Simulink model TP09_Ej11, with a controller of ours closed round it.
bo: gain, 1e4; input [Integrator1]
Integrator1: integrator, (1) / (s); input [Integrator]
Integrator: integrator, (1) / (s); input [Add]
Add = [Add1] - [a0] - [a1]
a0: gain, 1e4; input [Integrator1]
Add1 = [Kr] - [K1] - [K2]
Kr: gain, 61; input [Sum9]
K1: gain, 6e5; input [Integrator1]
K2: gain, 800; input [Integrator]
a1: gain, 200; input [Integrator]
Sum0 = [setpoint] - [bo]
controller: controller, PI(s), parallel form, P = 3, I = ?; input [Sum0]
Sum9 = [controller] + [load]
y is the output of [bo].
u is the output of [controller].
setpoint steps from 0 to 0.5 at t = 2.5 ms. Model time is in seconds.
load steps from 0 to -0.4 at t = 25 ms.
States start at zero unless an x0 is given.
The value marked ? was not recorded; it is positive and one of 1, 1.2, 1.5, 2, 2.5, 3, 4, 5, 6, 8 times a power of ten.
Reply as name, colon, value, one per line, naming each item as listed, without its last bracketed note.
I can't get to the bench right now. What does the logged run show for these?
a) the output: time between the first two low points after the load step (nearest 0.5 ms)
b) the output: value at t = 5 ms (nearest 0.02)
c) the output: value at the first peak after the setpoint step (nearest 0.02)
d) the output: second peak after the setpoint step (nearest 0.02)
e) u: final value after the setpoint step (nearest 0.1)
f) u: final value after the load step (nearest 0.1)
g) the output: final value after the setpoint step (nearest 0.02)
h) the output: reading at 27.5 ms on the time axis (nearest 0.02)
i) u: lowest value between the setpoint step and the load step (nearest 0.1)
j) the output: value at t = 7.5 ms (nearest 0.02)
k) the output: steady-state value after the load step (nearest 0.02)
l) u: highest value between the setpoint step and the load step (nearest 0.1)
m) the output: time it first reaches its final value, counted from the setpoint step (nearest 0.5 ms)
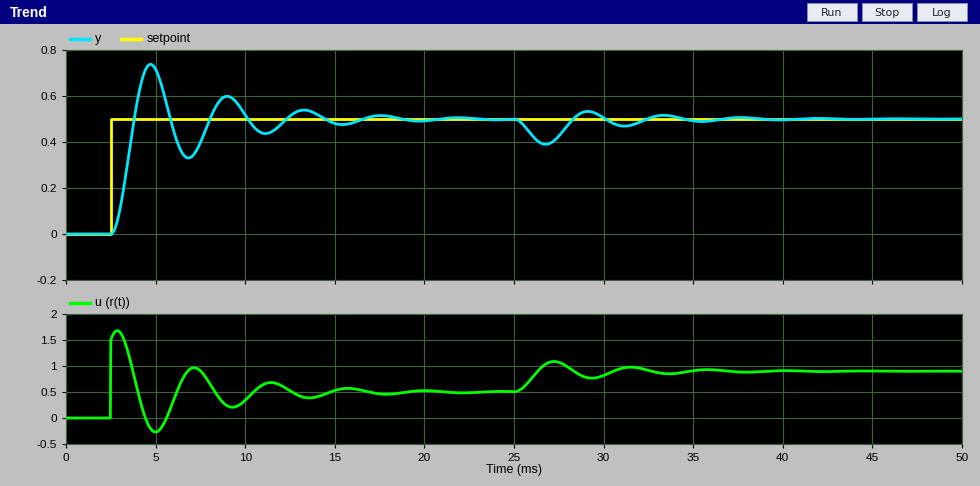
the output: time between the first two low points after the load step: 4.5 ms
the output: value at t = 5 ms: 0.72
the output: value at the first peak after the setpoint step: 0.74
the output: second peak after the setpoint step: 0.60
u: final value after the setpoint step: 0.5
u: final value after the load step: 0.9
the output: final value after the setpoint step: 0.50
the output: reading at 27.5 ms on the time axis: 0.42
u: lowest value between the setpoint step and the load step: -0.3
the output: value at t = 7.5 ms: 0.40
the output: steady-state value after the load step: 0.50
u: highest value between the setpoint step and the load step: 1.7
the output: time it first reaches its final value, counted from the setpoint step: 1.5 ms
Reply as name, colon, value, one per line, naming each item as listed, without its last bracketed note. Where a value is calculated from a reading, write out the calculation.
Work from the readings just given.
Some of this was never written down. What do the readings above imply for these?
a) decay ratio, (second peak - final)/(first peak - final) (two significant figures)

decay ratio, (second peak - final)/(first peak - final): (0.6 - 0.5) / (0.74 - 0.5) = 0.42
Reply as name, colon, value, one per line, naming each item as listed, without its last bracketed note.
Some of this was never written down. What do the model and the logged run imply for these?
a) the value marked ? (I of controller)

the value marked ?: 2000
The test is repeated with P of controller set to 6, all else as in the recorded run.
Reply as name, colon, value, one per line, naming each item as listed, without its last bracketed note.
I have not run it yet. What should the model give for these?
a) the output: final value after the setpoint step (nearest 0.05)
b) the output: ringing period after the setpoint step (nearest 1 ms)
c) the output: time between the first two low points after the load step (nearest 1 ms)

the output: final value after the setpoint step: 0.50
the output: ringing period after the setpoint step: 3 ms
the output: time between the first two low points after the load step: 3 ms
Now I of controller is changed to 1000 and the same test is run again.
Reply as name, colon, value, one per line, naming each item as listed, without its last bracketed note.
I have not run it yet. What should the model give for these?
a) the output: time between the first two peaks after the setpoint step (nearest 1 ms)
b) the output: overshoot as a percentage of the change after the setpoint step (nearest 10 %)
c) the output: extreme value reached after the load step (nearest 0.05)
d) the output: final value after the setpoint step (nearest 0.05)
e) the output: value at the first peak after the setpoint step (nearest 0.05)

the output: time between the first two peaks after the setpoint step: 4 ms
the output: overshoot as a percentage of the change after the setpoint step: 30 %
the output: extreme value reached after the load step: 0.40
the output: final value after the setpoint step: 0.50
the output: value at the first peak after the setpoint step: 0.65
